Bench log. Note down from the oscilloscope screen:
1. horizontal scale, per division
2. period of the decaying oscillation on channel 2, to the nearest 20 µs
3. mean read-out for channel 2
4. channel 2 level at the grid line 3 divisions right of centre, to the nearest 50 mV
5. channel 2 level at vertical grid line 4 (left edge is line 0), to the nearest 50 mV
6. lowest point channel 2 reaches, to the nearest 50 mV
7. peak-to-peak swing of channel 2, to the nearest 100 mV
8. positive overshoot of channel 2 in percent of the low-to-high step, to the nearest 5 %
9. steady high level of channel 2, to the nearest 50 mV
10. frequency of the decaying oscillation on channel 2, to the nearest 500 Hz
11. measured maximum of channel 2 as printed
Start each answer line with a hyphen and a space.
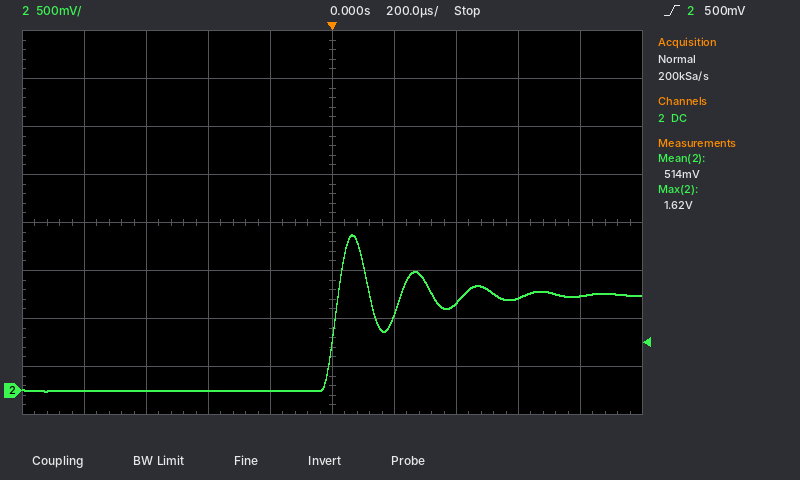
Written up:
- 200 µs
- 200 µs
- 514 mV
- 950 mV
- 0 mV
- 0 mV
- 1.60 V
- 60 %
- 1.00 V
- 5.0 kHz
- 1.62 V
